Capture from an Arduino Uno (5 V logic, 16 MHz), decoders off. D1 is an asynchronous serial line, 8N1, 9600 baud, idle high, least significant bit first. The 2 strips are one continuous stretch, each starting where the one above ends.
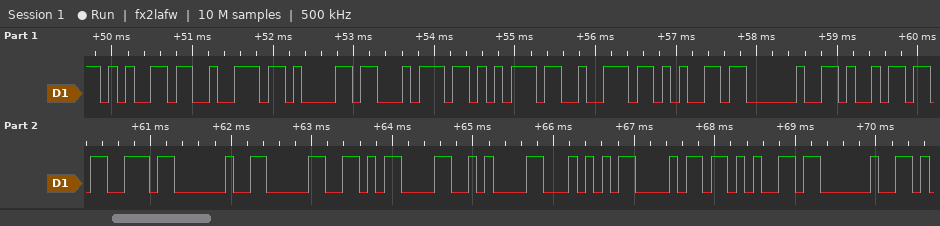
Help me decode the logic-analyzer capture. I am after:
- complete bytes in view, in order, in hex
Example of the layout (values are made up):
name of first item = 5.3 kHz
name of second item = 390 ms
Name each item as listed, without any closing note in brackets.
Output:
complete bytes in view, in order, in hex = 0x65 0x72 0x61 0x74 0x75 0x72 0x65 0x20 0x69 0x73 0x20 0x30 0x0D 0x0A 0x54 0x68 0x65 0x20
